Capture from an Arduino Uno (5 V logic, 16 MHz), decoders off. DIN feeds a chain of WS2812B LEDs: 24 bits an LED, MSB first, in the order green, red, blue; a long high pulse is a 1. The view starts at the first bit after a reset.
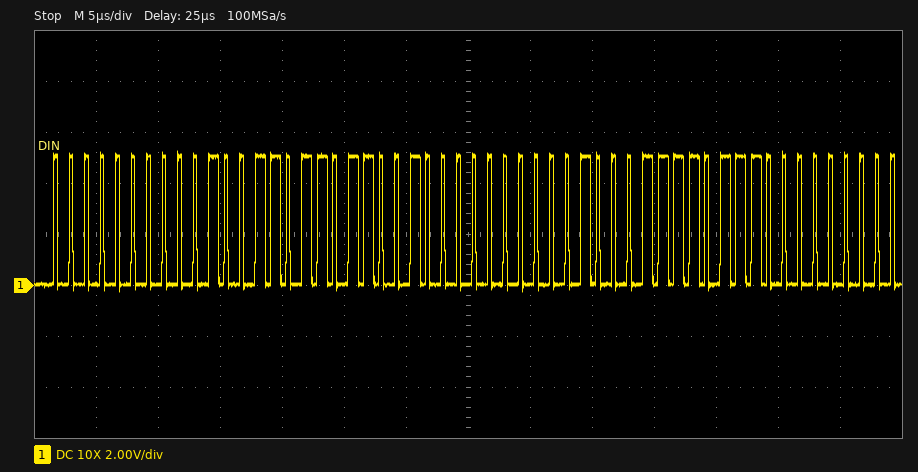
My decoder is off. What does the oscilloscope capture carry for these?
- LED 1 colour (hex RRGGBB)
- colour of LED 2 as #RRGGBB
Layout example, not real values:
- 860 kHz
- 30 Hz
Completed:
- #2600D9
- #2300DC
